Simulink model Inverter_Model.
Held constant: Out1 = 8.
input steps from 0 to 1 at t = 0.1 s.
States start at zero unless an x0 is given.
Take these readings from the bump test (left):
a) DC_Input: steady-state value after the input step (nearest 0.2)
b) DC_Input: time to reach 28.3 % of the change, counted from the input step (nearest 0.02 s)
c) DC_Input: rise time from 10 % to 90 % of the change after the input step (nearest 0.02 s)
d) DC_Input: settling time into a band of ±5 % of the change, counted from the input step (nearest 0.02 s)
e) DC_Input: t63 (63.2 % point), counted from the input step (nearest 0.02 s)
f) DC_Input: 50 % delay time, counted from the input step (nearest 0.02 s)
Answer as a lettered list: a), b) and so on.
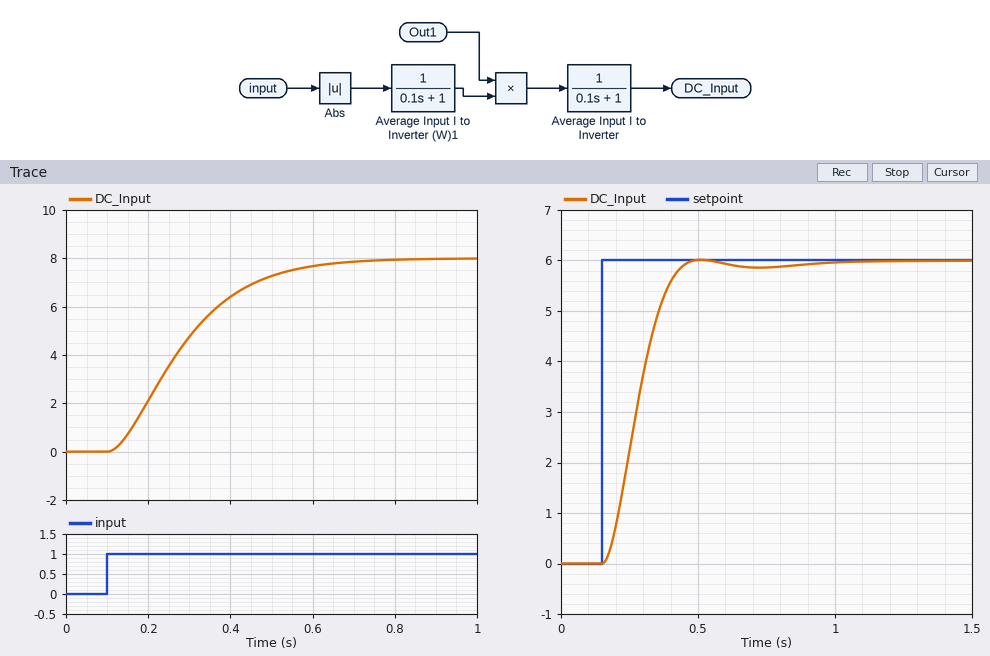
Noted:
a) 8.0
b) 0.10 s
c) 0.34 s
d) 0.48 s
e) 0.22 s
f) 0.16 s
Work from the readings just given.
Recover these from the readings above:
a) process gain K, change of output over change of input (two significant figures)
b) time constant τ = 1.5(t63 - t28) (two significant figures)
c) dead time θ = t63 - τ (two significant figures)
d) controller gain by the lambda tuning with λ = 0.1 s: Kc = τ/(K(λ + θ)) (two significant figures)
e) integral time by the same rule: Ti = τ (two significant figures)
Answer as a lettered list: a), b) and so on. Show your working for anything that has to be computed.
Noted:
a) (8 - 0) / 1 = 8.0
b) 1.5 × (0.22 - 0.1) = 0.18 s
c) 0.22 - 0.18 = 0.040 s
d) 0.18 / (8 × (0.1 + 0.04)) = 0.16
e) 0.18 s
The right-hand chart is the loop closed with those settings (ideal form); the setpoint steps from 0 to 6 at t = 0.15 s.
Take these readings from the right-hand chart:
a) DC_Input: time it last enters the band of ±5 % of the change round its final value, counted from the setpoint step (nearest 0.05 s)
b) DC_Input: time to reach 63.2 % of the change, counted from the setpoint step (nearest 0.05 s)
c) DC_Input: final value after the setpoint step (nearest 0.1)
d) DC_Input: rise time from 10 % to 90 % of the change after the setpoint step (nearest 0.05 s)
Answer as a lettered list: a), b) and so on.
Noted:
a) 0.25 s
b) 0.15 s
c) 6.0
d) 0.20 s
